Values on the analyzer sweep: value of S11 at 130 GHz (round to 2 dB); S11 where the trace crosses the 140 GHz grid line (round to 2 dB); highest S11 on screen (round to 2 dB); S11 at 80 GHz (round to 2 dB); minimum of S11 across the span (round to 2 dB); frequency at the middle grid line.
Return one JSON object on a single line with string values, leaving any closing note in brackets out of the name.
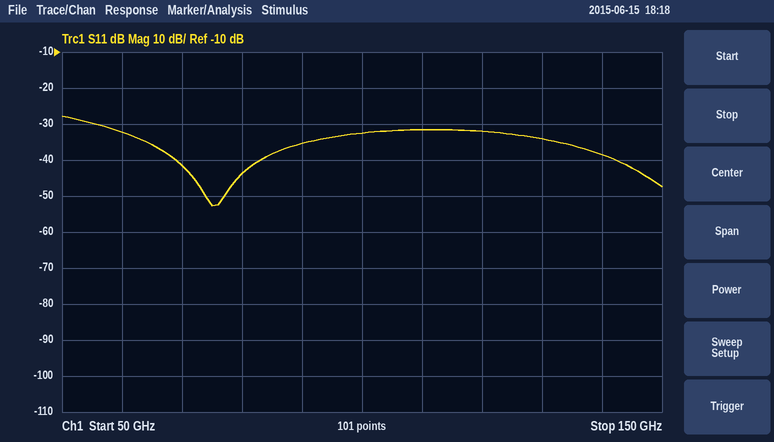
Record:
{"value of S11 at 130 GHz": "-34 dB", "S11 where the trace crosses the 140 GHz grid line": "-38 dB", "highest S11 on screen": "-28 dB", "S11 at 80 GHz": "-44 dB", "minimum of S11 across the span": "-52 dB", "frequency at the middle grid line": "100 GHz"}
